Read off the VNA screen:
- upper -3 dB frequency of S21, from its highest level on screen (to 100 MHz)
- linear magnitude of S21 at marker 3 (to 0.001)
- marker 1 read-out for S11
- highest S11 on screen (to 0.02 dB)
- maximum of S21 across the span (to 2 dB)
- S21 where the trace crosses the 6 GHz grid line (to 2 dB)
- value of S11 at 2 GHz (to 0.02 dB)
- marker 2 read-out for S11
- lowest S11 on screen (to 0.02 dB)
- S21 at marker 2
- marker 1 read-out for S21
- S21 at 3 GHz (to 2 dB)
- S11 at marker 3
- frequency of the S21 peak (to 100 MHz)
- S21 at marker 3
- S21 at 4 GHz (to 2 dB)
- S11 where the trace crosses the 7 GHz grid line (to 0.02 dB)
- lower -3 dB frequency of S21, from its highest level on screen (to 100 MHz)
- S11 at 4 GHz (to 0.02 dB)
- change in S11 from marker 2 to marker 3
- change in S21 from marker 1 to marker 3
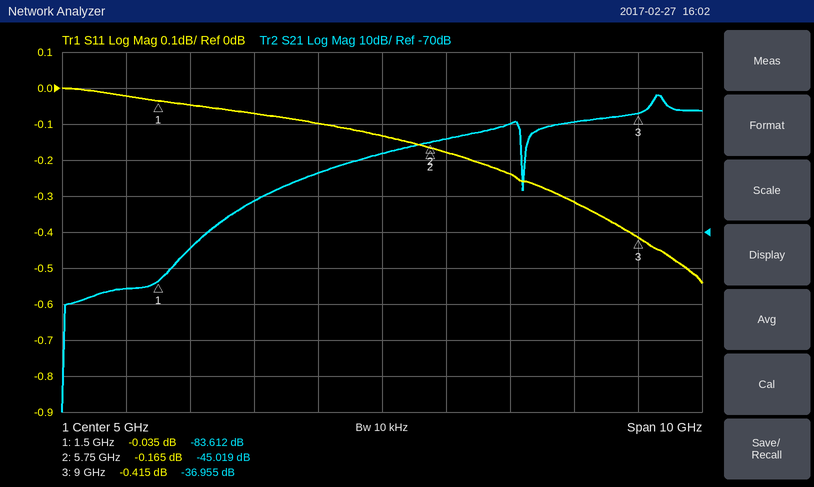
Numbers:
9.5 GHz
0.014
-0.035 dB
0.00 dB
-32 dB
-44 dB
-0.04 dB
-0.165 dB
-0.54 dB
-45.019 dB
-83.612 dB
-62 dB
-0.415 dB
9.3 GHz
-36.955 dB
-54 dB
-0.24 dB
9.2 GHz
-0.10 dB
-0.250 dB
46.657 dB
